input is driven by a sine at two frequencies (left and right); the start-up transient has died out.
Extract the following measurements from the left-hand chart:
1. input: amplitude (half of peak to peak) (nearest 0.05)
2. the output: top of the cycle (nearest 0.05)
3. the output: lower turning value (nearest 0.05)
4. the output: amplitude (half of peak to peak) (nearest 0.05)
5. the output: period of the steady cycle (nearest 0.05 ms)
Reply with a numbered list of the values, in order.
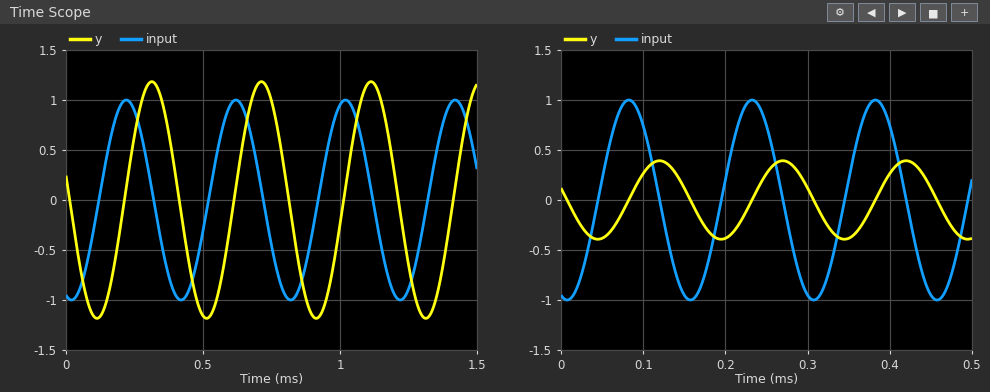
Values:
1. 1.00
2. 1.20
3. -1.20
4. 1.20
5. 0.40 ms
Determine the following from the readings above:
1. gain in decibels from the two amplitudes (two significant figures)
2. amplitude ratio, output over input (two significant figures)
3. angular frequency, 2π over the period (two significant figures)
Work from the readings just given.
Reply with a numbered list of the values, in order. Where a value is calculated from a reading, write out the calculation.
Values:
1. 20 log10(1.2 / 1) = 1.6 dB
2. 1.2 / 1 = 1.2
3. 2π / 0.4 = 16 rad/ms
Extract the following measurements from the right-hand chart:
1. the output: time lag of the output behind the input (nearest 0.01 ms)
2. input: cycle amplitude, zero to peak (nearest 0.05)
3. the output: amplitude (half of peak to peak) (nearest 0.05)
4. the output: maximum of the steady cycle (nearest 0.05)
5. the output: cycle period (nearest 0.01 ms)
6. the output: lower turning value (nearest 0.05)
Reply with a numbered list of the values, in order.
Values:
1. 0.04 ms
2. 1.00
3. 0.40
4. 0.40
5. 0.15 ms
6. -0.40
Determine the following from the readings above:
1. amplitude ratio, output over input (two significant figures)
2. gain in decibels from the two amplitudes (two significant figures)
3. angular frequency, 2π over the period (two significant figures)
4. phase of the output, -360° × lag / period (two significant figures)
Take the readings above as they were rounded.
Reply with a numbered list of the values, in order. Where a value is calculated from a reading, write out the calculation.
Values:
1. 0.4 / 1 = 0.40
2. 20 log10(0.4 / 1) = -8.0 dB
3. 2π / 0.15 = 42 rad/ms
4. -360 × 0.04 / 0.15 = -96°
